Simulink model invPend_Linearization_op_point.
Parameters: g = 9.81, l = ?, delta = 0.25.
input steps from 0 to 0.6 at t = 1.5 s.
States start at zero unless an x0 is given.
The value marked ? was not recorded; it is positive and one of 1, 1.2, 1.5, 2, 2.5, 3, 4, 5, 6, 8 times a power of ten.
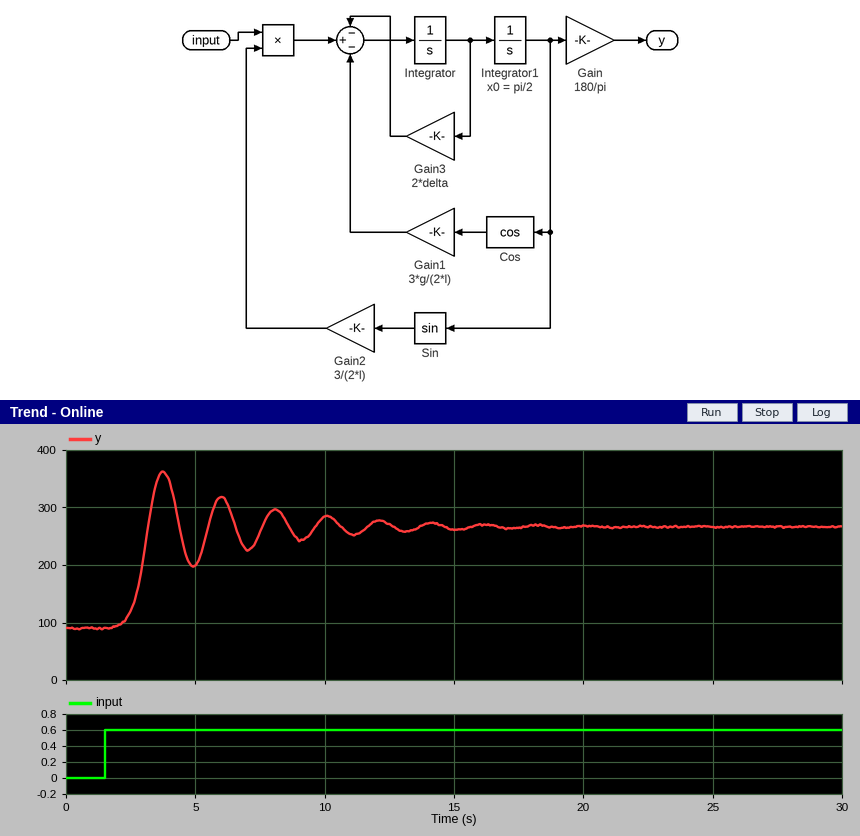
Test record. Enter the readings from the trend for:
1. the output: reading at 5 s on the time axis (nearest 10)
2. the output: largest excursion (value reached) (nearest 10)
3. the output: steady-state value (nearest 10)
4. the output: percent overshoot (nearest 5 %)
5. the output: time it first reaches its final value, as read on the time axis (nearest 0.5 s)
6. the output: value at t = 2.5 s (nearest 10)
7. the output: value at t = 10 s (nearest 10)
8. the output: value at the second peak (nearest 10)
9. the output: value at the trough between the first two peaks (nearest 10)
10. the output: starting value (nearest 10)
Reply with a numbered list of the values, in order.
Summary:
1. 200
2. 360
3. 270
4. 55 %
5. 3.0 s
6. 120
7. 280
8. 320
9. 200
10. 90
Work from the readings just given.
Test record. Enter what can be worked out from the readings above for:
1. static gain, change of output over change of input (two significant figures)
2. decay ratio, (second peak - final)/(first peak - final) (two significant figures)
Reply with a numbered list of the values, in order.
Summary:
1. 300
2. 0.56
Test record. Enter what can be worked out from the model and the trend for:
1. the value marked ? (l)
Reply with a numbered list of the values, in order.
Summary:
1. 1.5
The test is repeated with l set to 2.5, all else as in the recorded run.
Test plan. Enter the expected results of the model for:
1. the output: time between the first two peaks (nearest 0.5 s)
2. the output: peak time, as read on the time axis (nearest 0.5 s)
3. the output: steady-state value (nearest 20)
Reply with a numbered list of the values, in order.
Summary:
1. 3.0 s
2. 4.5 s
3. 260
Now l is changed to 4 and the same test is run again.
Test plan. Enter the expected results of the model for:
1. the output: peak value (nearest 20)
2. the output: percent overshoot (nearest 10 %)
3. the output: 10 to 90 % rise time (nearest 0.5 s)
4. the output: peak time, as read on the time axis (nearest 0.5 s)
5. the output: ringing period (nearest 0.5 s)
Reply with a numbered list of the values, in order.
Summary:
1. 340
2. 40 %
3. 1.5 s
4. 5.0 s
5. 3.5 s
